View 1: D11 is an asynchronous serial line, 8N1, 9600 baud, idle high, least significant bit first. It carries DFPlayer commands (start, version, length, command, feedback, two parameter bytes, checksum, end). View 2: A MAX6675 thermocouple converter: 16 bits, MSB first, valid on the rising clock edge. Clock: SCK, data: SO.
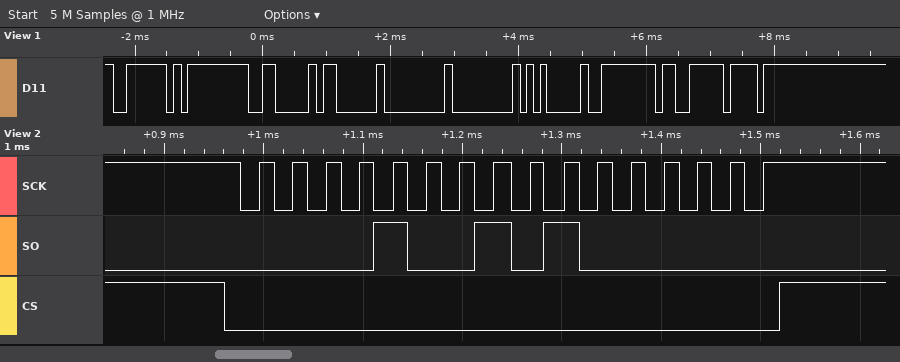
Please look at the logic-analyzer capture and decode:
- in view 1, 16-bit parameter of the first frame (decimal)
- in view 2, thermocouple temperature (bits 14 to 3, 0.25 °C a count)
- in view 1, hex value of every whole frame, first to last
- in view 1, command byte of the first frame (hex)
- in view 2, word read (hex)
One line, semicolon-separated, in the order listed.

5; 74.00 °C; 7E FF 06 03 00 00 05 FE F3 EF; 0x03; 0x0940
